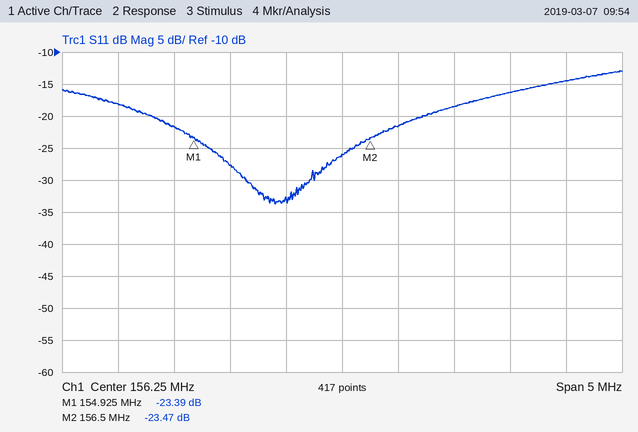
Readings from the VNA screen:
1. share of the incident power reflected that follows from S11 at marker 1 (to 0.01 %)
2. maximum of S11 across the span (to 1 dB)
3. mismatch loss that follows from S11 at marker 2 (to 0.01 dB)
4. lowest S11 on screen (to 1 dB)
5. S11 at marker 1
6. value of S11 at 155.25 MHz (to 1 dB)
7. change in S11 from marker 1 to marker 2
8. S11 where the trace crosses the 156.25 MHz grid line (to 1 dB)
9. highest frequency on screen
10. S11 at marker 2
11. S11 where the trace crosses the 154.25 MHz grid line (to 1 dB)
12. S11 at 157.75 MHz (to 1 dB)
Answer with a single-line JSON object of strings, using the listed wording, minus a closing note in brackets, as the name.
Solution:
{"share of the incident power reflected that follows from S11 at marker 1": "0.46 %", "maximum of S11 across the span": "-13 dB", "mismatch loss that follows from S11 at marker 2": "0.02 dB", "lowest S11 on screen": "-34 dB", "S11 at marker 1": "-23.39 dB", "value of S11 at 155.25 MHz": "-28 dB", "change in S11 from marker 1 to marker 2": "-0.08 dB", "S11 where the trace crosses the 156.25 MHz grid line": "-26 dB", "highest frequency on screen": "158.75 MHz", "S11 at marker 2": "-23.47 dB", "S11 where the trace crosses the 154.25 MHz grid line": "-18 dB", "S11 at 157.75 MHz": "-16 dB"}
